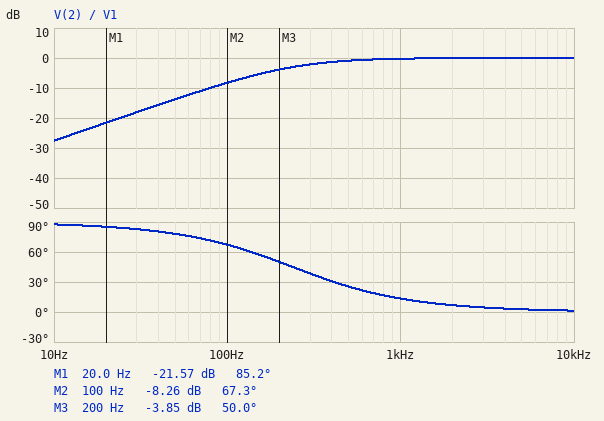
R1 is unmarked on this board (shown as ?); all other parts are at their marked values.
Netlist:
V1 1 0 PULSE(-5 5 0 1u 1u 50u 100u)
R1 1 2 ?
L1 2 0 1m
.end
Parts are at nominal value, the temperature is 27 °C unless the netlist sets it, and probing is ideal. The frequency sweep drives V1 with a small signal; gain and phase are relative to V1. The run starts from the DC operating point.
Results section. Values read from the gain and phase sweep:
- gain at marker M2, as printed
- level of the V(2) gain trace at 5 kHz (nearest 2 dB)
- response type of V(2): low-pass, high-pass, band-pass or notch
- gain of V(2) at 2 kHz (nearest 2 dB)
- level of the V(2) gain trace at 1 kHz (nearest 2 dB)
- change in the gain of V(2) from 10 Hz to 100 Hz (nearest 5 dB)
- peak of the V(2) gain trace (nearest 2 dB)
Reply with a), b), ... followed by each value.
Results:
a) -8.26 dB
b) 0 dB
c) high-pass
d) 0 dB
e) 0 dB
f) 20 dB
g) 0 dB
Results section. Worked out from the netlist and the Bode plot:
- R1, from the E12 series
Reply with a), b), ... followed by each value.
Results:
a) 1.5 Ω
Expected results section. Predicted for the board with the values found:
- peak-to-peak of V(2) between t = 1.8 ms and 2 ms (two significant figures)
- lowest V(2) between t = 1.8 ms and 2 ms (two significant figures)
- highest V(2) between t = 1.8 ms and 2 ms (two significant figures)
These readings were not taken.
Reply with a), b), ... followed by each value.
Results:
a) 10 V
b) -5.0 V
c) 5.4 V
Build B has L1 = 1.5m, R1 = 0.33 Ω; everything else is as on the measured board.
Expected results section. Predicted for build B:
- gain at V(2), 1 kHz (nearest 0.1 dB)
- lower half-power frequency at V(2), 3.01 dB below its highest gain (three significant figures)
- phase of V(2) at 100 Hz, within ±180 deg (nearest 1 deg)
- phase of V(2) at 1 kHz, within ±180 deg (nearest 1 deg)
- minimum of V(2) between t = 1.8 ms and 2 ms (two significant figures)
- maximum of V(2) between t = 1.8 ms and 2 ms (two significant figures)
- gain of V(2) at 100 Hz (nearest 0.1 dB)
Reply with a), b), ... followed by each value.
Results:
a) 0 dB
b) 35.0 Hz
c) 19 deg
d) 2 deg
e) -1.8 V
f) 8.3 V
g) -0.5 dB
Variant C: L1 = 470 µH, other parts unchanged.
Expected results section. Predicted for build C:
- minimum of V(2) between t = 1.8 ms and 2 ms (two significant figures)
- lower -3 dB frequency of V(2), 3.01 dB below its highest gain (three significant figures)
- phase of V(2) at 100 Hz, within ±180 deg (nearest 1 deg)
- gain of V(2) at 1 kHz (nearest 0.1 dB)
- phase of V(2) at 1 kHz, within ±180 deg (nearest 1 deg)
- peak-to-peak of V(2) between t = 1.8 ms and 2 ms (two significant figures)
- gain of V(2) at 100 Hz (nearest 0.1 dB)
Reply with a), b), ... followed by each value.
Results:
a) -5.5 V
b) 508 Hz
c) 79 deg
d) -1.0 dB
e) 27 deg
f) 11 V
g) -14.3 dB
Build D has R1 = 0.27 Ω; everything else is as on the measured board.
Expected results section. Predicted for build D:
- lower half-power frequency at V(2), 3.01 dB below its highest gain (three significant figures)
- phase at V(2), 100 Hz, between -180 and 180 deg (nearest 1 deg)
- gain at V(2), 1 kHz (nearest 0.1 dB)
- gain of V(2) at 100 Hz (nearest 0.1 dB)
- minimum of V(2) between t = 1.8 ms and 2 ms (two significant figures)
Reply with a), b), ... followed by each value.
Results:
a) 43.0 Hz
b) 23 deg
c) 0 dB
d) -0.7 dB
e) -2.1 V
